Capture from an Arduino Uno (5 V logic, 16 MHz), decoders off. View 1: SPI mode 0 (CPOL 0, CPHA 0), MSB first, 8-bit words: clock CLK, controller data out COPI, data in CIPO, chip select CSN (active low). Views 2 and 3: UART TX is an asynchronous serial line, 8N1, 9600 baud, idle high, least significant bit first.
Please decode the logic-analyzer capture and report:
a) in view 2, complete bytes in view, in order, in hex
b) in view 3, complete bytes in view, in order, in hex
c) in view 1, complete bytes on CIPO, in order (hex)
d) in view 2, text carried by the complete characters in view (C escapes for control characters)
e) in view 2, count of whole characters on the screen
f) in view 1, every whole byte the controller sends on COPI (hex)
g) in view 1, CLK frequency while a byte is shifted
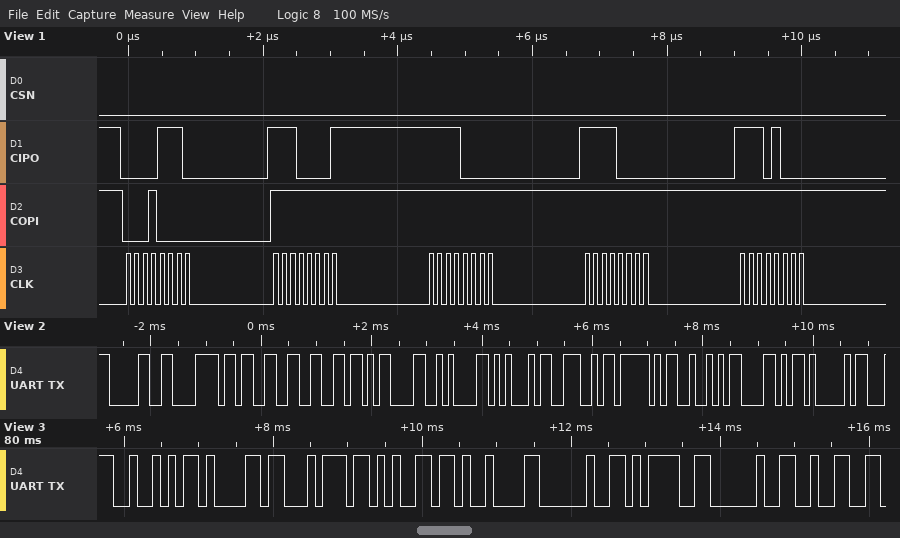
0x30 0x78 0x33 0x66 0x0D 0x0A 0x45 0x4E 0x5F 0x52 0x58 0x41
52 61 74 65 09 20 3D 20 32
0E E1 F0 F0 E8
"0x3f\r\nEN_RXA"
12
10 FF FF FF FF
8 MHz
